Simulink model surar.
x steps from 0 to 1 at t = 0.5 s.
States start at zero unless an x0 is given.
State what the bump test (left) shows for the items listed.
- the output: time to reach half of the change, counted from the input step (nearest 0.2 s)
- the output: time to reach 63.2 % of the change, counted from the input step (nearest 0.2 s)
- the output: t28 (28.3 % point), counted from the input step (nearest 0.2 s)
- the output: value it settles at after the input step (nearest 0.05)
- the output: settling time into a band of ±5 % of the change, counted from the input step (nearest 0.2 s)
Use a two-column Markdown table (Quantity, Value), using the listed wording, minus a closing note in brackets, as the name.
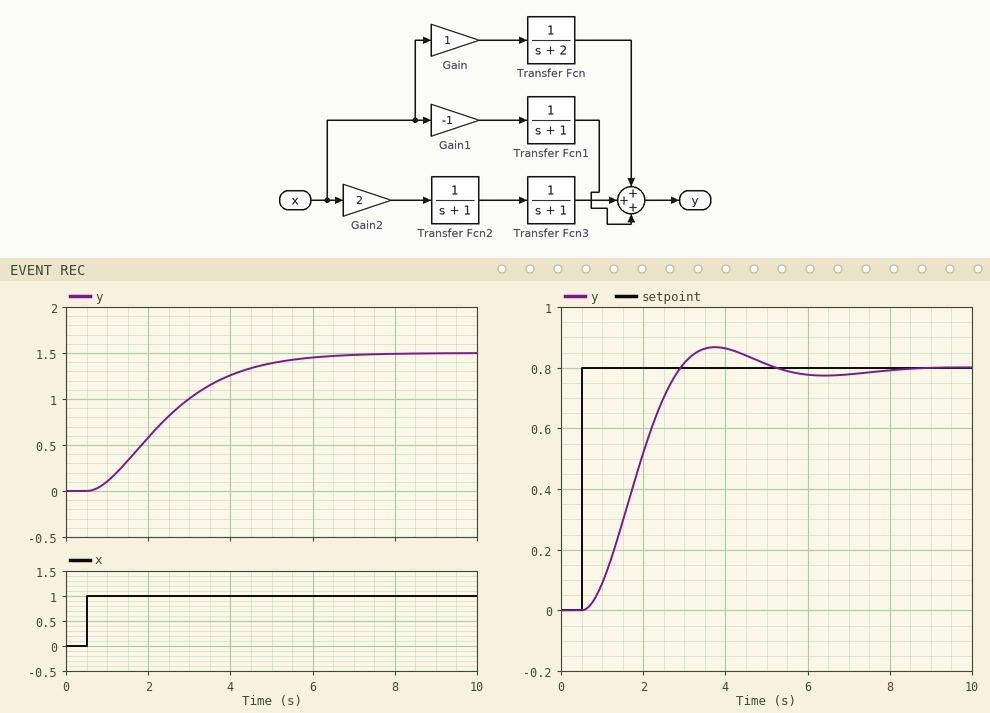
| Quantity | Value |
|---|---|
| the output: time to reach half of the change, counted from the input step | 1.8 s |
| the output: time to reach 63.2 % of the change, counted from the input step | 2.4 s |
| the output: t28 (28.3 % point), counted from the input step | 1.2 s |
| the output: value it settles at after the input step | 1.50 |
| the output: settling time into a band of ±5 % of the change, counted from the input step | 5.0 s |
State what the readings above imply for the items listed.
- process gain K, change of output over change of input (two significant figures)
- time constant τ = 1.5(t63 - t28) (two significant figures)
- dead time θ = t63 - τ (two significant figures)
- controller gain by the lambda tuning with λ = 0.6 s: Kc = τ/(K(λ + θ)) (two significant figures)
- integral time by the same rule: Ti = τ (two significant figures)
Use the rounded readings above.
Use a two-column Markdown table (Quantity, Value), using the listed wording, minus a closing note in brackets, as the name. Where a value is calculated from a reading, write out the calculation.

| Quantity | Value |
|---|---|
| process gain K, change of output over change of input | (1.5 - 0) / 1 = 1.5 |
| time constant τ = 1.5(t63 - t28) | 1.5 × (2.4 - 1.2) = 1.8 s |
| dead time θ = t63 - τ | 2.4 - 1.8 = 0.60 s |
| controller gain by the lambda tuning with λ = 0.6 s: Kc = τ/(K(λ + θ)) | 1.8 / (1.5 × (0.6 + 0.6)) = 1.0 |
| integral time by the same rule: Ti = τ | 1.8 s |
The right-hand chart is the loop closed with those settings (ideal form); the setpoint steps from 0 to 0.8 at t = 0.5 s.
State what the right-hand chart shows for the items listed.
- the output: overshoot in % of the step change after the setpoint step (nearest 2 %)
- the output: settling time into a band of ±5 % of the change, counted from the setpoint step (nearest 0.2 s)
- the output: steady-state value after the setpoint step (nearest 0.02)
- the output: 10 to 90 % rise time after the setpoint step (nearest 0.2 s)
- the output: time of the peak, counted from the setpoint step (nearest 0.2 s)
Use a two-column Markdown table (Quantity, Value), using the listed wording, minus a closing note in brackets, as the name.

| Quantity | Value |
|---|---|
| the output: overshoot in % of the step change after the setpoint step | 8 % |
| the output: settling time into a band of ±5 % of the change, counted from the setpoint step | 4.0 s |
| the output: steady-state value after the setpoint step | 0.80 |
| the output: 10 to 90 % rise time after the setpoint step | 1.6 s |
| the output: time of the peak, counted from the setpoint step | 3.2 s |
